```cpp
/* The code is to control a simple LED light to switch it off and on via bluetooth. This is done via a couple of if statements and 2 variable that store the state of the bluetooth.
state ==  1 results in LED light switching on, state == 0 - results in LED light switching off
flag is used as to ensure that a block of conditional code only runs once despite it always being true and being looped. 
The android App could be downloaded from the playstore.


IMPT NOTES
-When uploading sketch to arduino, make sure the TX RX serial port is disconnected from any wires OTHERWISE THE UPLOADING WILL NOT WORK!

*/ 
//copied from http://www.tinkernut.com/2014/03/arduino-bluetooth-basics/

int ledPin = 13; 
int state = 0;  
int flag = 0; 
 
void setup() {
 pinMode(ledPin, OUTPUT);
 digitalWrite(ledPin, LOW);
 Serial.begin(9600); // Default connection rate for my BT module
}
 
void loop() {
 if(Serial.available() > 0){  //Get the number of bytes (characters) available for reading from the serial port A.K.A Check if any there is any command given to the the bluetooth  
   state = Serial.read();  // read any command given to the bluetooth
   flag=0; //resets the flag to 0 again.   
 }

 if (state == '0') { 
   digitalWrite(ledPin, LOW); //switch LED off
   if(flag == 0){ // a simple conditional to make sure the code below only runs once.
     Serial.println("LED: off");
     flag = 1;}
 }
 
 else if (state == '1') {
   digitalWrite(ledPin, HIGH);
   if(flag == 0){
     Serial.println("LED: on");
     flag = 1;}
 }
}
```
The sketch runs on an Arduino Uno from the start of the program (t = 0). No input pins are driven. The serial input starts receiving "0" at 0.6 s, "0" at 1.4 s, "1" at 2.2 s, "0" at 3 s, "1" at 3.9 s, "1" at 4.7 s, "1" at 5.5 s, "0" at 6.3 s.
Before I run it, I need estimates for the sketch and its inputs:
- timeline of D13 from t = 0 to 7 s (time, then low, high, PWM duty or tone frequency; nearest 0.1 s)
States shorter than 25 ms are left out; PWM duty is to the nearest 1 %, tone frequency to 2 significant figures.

0 s low; 2.2 s high; 3 s low; 3.9 s high; 6.3 s low
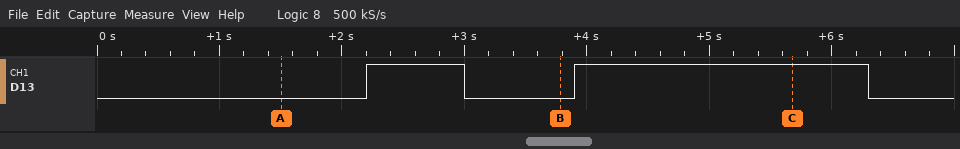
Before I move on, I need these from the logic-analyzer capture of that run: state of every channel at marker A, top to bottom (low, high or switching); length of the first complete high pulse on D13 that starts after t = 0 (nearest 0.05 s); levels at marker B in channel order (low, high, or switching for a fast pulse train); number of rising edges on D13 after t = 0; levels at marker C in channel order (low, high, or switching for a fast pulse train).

D13 low
0.80 s
D13 low
2
D13 high
